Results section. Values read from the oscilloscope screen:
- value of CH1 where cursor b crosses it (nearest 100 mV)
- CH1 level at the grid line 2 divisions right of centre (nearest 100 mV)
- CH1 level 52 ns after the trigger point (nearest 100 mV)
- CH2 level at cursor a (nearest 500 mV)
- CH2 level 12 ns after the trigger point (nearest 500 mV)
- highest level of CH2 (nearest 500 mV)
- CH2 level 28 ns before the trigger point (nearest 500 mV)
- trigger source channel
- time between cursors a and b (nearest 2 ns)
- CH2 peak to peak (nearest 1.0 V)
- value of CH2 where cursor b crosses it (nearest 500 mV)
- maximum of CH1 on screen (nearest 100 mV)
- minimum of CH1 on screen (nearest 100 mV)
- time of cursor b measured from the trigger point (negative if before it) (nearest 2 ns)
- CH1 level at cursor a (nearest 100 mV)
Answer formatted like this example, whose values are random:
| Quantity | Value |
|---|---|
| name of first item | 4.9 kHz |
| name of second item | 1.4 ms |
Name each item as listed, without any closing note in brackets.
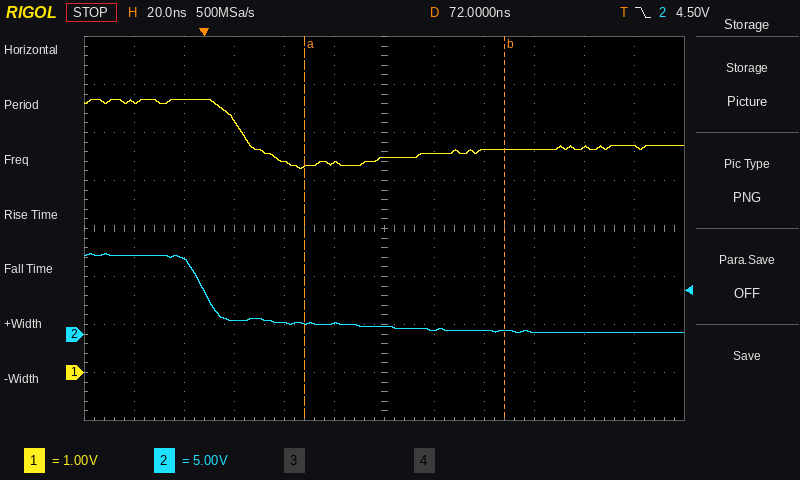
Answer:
| Quantity | Value |
|---|---|
| value of CH1 where cursor b crosses it | 4.6 V |
| CH1 level at the grid line 2 divisions right of centre | 4.6 V |
| CH1 level 52 ns after the trigger point | 4.4 V |
| CH2 level at cursor a | 1.0 V |
| CH2 level 12 ns after the trigger point | 1.5 V |
| highest level of CH2 | 8.5 V |
| CH2 level 28 ns before the trigger point | 8.0 V |
| trigger source channel | CH2 |
| time between cursors a and b | 80 ns |
| CH2 peak to peak | 8.0 V |
| value of CH2 where cursor b crosses it | 500 mV |
| maximum of CH1 on screen | 5.7 V |
| minimum of CH1 on screen | 4.2 V |
| time of cursor b measured from the trigger point (negative if before it) | +120 ns |
| CH1 level at cursor a | 4.3 V |
